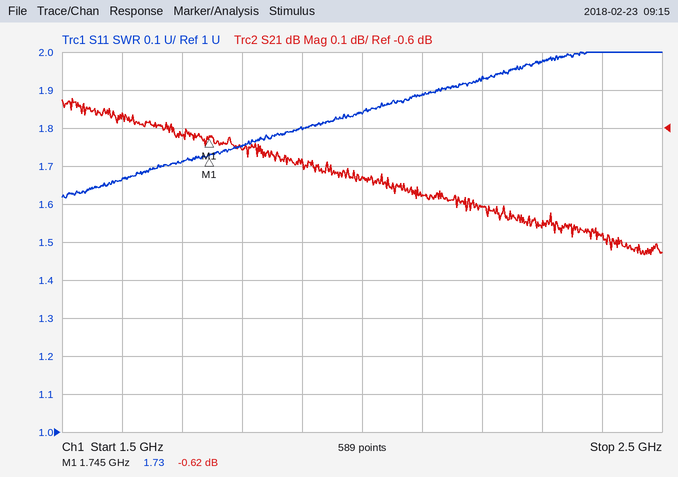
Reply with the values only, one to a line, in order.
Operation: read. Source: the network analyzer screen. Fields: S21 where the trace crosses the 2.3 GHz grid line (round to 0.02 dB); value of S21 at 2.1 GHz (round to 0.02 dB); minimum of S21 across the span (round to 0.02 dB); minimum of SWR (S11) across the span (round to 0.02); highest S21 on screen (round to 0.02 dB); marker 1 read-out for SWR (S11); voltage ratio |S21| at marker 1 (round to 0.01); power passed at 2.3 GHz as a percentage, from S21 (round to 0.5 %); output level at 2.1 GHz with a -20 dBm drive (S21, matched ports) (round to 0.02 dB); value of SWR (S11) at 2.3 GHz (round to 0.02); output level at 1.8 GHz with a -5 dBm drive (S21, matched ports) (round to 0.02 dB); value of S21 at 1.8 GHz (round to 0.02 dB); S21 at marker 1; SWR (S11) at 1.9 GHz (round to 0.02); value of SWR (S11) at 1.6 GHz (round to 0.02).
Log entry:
-0.86 dB
-0.78 dB
-0.94 dB
1.62
-0.52 dB
1.73
0.93
82.0 %
-20.78 dBm
1.98
-5.66 dBm
-0.66 dB
-0.62 dB
1.80
1.66
